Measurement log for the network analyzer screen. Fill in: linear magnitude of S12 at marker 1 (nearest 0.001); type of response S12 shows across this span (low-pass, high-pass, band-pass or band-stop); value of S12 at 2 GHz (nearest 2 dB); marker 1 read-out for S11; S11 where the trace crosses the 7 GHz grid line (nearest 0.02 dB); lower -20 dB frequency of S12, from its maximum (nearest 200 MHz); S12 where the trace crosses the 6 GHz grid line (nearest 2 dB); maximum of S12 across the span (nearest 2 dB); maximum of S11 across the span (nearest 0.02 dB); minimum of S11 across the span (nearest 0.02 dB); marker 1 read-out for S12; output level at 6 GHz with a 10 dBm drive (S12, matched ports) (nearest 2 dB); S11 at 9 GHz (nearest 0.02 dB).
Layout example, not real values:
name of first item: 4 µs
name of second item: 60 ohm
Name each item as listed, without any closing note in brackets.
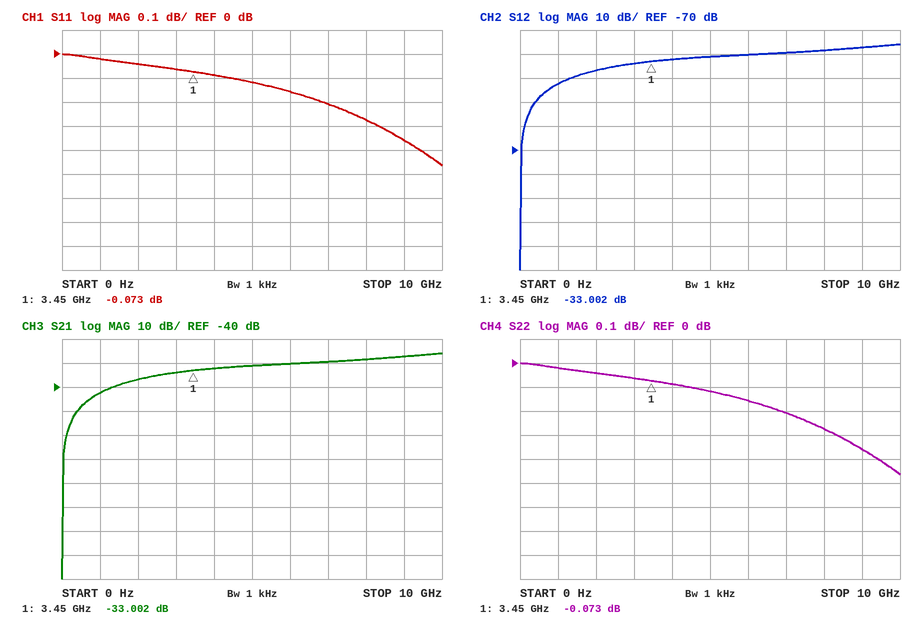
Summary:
linear magnitude of S12 at marker 1: 0.022
type of response S12 shows across this span: high-pass
value of S12 at 2 GHz: -36 dB
marker 1 read-out for S11: -0.073 dB
S11 where the trace crosses the 7 GHz grid line: -0.20 dB
lower -20 dB frequency of S12, from its maximum: 600 MHz
S12 where the trace crosses the 6 GHz grid line: -30 dB
maximum of S12 across the span: -26 dB
maximum of S11 across the span: 0.00 dB
minimum of S11 across the span: -0.46 dB
marker 1 read-out for S12: -33.002 dB
output level at 6 GHz with a 10 dBm drive (S12, matched ports): -20 dBm
S11 at 9 GHz: -0.36 dB
